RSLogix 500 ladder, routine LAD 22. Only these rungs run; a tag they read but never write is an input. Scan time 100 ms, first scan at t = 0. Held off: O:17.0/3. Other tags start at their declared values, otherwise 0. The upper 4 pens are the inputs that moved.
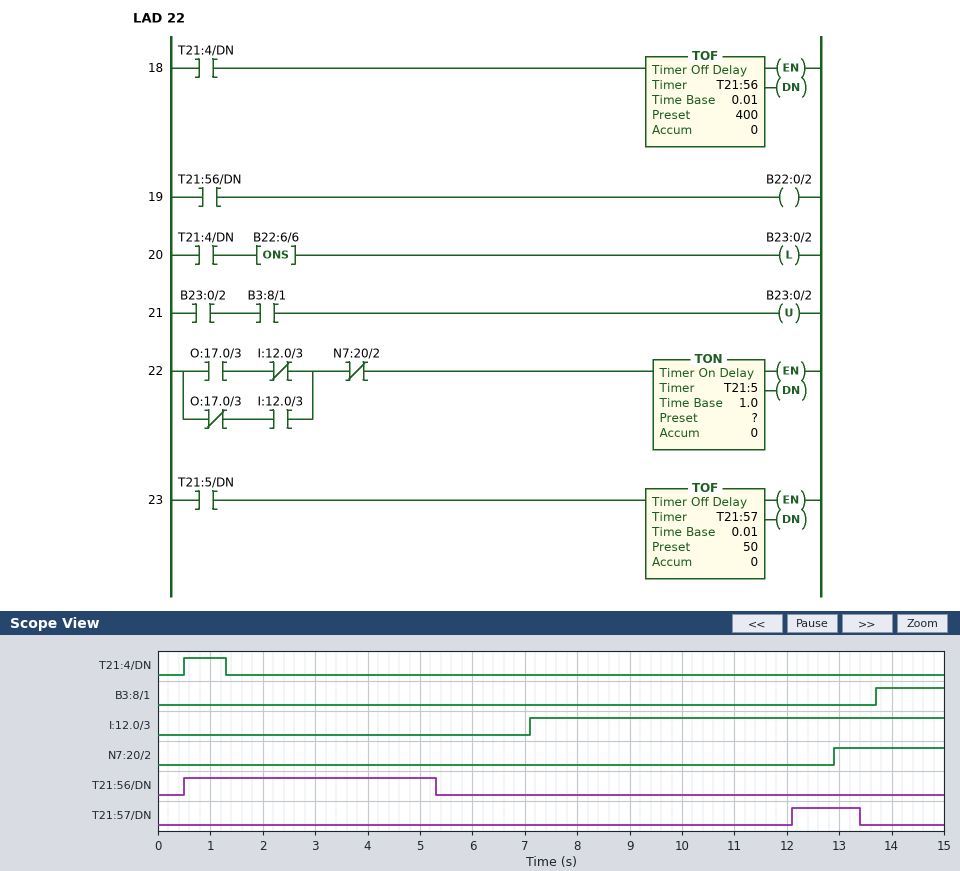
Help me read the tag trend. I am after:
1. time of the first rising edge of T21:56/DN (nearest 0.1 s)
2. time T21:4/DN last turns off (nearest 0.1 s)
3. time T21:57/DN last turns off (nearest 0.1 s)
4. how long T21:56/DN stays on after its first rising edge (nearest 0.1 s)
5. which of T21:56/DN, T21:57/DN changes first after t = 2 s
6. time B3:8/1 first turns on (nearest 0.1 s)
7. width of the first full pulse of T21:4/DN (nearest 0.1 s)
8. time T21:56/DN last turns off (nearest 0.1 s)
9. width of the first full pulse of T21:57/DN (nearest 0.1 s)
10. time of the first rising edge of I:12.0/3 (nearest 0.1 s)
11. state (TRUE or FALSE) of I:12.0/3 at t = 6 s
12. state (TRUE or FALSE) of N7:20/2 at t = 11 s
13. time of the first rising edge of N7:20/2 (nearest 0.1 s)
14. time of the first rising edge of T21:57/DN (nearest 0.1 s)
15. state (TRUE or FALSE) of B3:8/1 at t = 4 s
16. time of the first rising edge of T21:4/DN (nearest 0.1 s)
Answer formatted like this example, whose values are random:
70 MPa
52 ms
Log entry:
0.5 s
1.3 s
13.4 s
4.8 s
T21:56/DN
13.7 s
0.8 s
5.3 s
1.3 s
7.1 s
FALSE
FALSE
12.9 s
12.1 s
FALSE
0.5 s
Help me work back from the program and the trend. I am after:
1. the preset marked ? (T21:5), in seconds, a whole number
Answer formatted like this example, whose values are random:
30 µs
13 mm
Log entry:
5 s
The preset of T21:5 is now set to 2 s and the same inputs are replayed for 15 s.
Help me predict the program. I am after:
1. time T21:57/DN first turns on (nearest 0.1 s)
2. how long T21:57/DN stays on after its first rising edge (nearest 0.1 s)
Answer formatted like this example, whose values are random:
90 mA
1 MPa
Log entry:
9.1 s
4.3 s
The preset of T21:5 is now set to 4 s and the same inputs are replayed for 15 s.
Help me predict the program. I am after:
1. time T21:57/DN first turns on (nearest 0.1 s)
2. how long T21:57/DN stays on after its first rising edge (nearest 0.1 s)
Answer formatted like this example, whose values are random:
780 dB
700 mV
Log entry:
11.1 s
2.3 s
